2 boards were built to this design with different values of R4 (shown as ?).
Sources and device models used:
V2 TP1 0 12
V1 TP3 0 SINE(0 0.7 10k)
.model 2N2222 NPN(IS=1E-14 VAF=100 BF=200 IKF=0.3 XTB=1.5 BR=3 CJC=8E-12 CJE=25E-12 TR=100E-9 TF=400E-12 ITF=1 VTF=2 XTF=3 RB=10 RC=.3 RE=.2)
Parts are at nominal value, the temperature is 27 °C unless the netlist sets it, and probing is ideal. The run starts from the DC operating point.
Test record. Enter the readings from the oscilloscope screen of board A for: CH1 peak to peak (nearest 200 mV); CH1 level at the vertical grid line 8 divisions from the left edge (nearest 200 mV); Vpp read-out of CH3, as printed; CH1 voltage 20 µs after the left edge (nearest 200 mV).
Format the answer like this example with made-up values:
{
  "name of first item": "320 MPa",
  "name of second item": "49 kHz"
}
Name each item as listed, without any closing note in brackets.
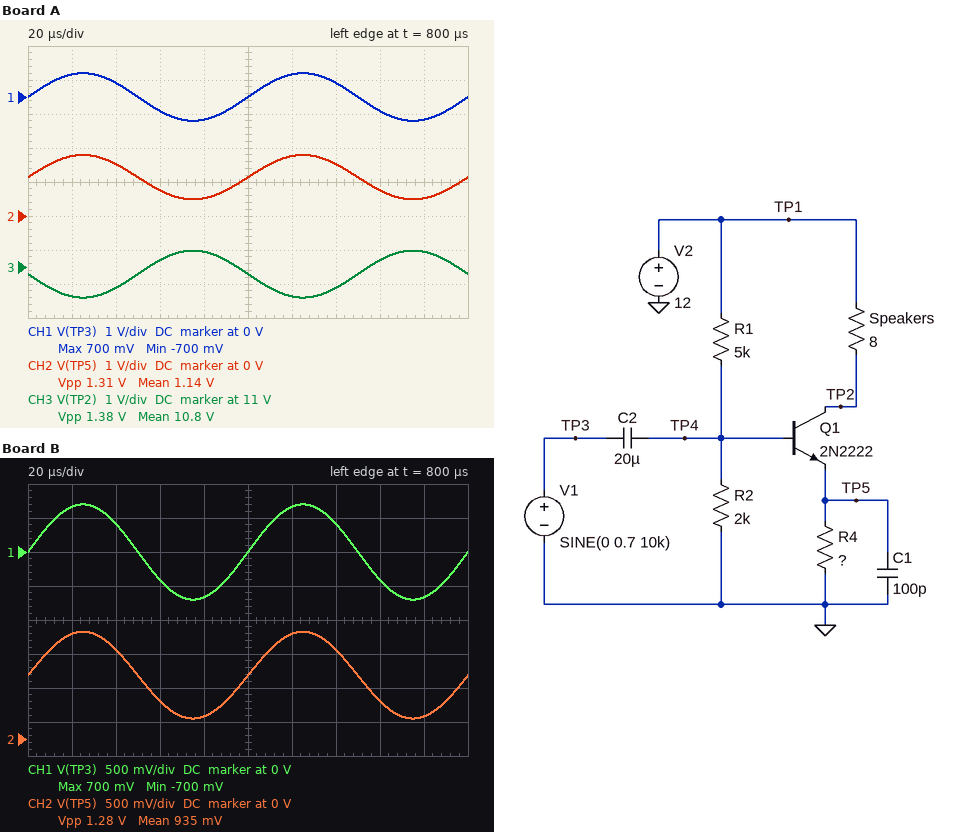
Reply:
{
  "CH1 peak to peak": "1.4 V",
  "CH1 level at the vertical grid line 8 divisions from the left edge": "-400 mV",
  "Vpp read-out of CH3, as printed": "1.38 V",
  "CH1 voltage 20 µs after the left edge": "600 mV"
}
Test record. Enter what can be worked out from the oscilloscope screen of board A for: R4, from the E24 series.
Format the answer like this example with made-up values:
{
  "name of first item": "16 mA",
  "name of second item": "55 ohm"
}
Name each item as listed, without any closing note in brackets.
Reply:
{
  "R4, from the E24 series": "7.5 Ω"
}
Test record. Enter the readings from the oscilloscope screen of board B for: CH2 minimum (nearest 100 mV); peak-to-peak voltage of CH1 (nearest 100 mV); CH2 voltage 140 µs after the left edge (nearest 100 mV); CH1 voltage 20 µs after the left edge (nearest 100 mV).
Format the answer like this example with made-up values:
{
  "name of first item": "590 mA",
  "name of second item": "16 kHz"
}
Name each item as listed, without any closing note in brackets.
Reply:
{
  "CH2 minimum": "300 mV",
  "peak-to-peak voltage of CH1": "1.4 V",
  "CH2 voltage 140 µs after the left edge": "1.3 V",
  "CH1 voltage 20 µs after the left edge": "700 mV"
}
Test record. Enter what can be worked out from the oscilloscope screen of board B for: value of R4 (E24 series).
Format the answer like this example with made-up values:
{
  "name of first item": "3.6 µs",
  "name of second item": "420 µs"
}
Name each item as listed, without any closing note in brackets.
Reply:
{
  "value of R4": "5.6 Ω"
}
